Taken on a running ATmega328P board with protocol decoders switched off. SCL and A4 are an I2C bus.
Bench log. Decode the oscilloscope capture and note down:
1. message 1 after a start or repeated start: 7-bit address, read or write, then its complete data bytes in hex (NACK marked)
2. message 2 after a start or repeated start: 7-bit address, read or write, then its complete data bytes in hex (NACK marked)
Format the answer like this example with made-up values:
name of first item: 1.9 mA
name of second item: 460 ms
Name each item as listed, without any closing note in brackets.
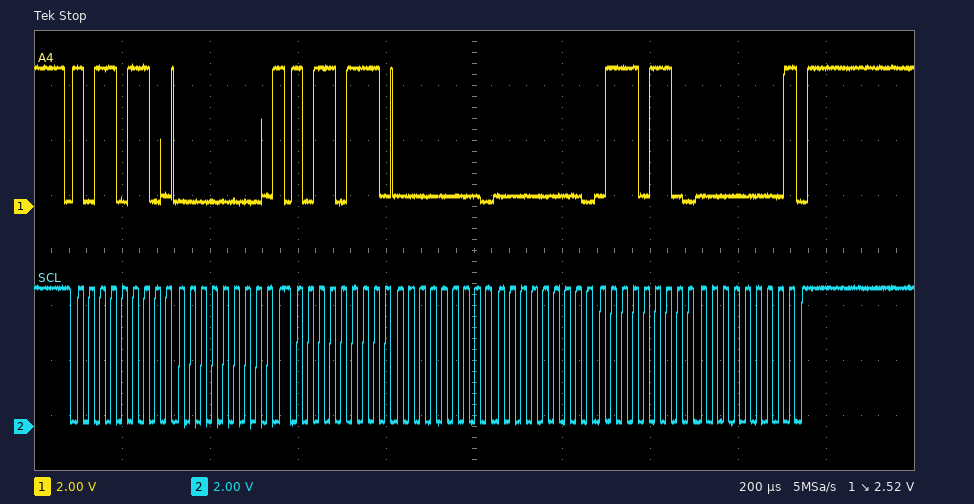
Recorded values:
message 1 after a start or repeated start: 7-bit address, read or write, then its complete data bytes in hex: 0x5B write: 00
message 2 after a start or repeated start: 7-bit address, read or write, then its complete data bytes in hex: 0x5B read: 00 00 76 00 NACK
